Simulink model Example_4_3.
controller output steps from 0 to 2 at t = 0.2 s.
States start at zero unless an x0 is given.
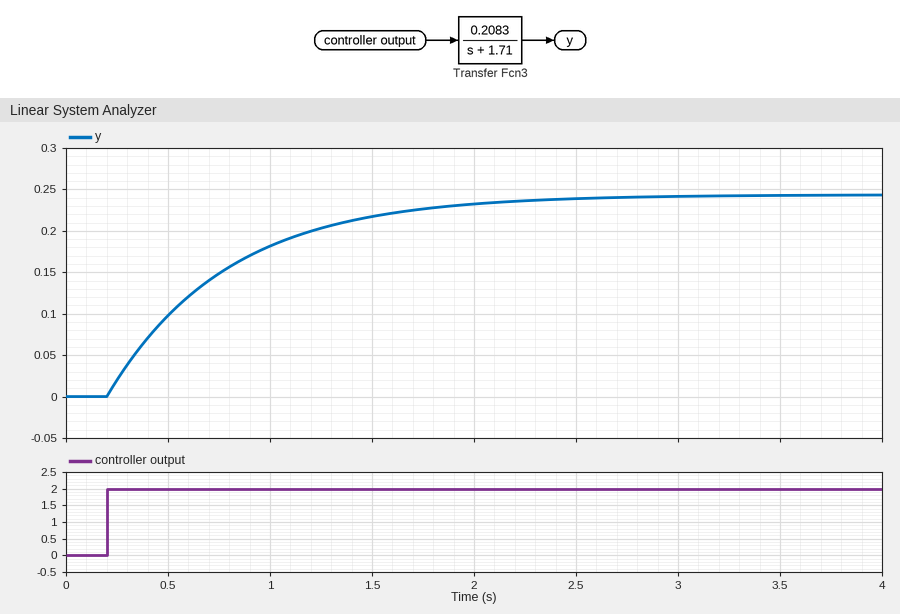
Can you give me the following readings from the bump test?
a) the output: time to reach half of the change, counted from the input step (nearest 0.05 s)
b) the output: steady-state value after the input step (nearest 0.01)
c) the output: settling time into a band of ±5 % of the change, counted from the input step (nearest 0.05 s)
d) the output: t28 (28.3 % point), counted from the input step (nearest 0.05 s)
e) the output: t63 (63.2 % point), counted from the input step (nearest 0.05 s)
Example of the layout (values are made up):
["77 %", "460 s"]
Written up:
["0.40 s", "0.24", "1.75 s", "0.20 s", "0.60 s"]
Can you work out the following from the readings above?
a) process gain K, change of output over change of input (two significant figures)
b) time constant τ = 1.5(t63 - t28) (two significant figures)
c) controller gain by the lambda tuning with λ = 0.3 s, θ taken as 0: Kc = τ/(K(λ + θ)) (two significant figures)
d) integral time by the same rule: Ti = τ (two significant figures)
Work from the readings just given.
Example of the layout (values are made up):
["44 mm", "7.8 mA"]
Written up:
["0.12", "0.60 s", "17", "0.60 s"]
